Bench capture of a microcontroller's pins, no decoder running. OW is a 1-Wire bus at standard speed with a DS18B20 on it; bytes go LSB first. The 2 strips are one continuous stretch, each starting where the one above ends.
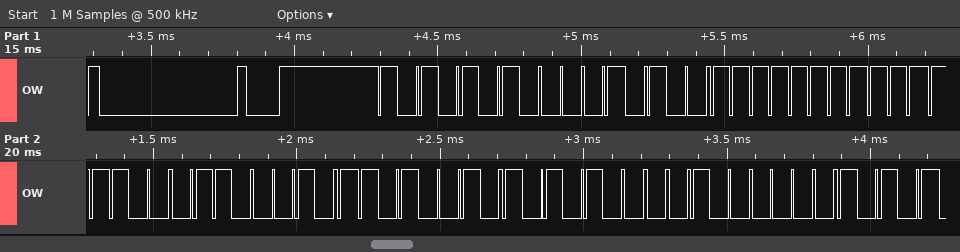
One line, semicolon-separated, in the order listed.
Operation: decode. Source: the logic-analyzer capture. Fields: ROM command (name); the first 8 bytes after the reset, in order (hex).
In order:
Match ROM; 55 28 FF 3F 46 4B 15 02
